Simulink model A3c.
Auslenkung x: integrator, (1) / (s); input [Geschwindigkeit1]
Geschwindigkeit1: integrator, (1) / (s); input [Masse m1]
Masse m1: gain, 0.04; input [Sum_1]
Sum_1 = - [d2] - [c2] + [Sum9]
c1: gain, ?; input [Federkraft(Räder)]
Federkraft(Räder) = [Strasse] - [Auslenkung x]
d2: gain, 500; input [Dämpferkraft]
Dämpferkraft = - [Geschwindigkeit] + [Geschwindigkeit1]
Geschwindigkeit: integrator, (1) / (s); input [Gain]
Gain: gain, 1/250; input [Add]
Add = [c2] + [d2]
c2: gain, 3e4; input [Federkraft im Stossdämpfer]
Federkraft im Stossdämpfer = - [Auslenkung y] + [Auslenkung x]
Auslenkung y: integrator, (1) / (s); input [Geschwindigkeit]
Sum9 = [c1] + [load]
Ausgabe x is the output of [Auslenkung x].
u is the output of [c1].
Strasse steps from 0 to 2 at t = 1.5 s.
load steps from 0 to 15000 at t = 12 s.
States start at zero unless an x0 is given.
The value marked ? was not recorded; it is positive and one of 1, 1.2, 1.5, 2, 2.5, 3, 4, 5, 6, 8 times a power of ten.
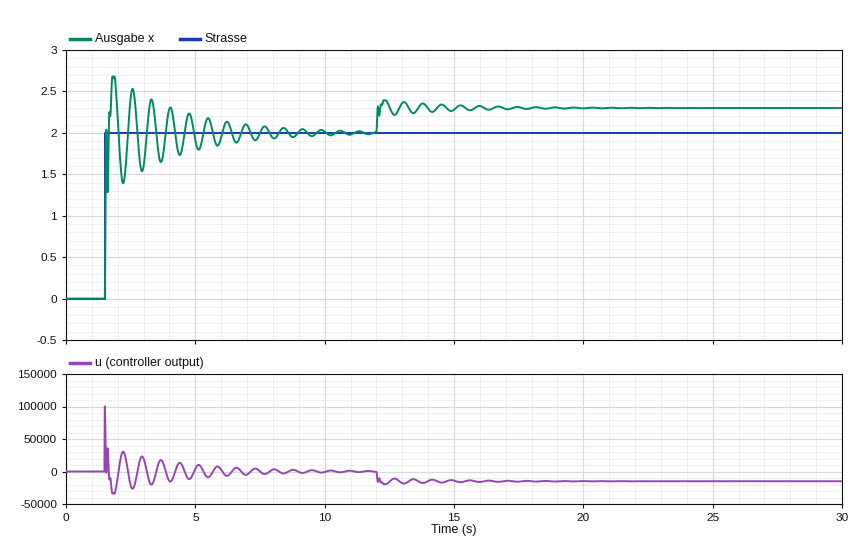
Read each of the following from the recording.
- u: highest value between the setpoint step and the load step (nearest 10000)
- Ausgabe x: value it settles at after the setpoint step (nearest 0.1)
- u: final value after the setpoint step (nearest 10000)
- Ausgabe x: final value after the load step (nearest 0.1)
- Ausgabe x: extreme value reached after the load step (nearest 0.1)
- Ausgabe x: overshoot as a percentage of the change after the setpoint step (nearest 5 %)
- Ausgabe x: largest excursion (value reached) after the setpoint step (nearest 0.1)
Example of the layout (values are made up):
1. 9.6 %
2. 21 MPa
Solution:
1. 100000
2. 2.0
3. 0
4. 2.3
5. 2.4
6. 35 %
7. 2.7
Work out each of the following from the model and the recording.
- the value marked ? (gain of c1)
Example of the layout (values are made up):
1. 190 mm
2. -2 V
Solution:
1. 50000
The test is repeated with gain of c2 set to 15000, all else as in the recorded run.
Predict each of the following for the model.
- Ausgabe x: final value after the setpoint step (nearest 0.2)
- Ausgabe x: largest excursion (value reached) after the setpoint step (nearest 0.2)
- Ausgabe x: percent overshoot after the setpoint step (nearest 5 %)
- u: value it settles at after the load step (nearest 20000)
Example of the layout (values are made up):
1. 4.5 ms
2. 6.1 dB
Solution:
1. 2.0
2. 2.4
3. 20 %
4. -20000
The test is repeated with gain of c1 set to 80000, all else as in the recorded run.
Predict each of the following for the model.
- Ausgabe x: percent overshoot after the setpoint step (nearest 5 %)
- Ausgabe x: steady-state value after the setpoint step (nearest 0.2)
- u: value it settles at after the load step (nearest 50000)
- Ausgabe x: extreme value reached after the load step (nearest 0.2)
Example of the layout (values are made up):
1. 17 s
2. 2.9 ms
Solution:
1. 25 %
2. 2.0
3. 0
4. 2.2
